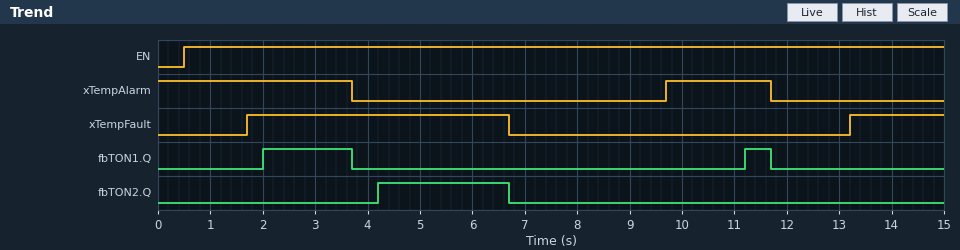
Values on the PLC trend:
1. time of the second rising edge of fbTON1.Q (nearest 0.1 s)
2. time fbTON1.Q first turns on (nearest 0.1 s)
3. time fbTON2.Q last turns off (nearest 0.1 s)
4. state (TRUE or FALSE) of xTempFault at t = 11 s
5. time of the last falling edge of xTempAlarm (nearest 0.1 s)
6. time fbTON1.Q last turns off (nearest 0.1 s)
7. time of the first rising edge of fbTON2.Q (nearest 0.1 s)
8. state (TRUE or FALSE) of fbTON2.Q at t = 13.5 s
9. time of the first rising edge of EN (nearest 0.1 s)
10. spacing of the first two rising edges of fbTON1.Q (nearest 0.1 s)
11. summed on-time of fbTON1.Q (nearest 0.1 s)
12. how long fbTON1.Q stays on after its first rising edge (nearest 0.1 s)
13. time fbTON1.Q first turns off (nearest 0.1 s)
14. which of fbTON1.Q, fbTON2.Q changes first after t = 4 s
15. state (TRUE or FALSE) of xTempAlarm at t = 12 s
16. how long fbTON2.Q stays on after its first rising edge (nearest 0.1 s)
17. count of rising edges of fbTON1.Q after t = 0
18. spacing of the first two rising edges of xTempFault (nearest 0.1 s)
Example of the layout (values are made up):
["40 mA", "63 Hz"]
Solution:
["11.2 s", "2.0 s", "6.7 s", "FALSE", "11.7 s", "11.7 s", "4.2 s", "FALSE", "0.5 s", "9.2 s", "2.2 s", "1.7 s", "3.7 s", "fbTON2.Q", "FALSE", "2.5 s", "2", "11.5 s"]
